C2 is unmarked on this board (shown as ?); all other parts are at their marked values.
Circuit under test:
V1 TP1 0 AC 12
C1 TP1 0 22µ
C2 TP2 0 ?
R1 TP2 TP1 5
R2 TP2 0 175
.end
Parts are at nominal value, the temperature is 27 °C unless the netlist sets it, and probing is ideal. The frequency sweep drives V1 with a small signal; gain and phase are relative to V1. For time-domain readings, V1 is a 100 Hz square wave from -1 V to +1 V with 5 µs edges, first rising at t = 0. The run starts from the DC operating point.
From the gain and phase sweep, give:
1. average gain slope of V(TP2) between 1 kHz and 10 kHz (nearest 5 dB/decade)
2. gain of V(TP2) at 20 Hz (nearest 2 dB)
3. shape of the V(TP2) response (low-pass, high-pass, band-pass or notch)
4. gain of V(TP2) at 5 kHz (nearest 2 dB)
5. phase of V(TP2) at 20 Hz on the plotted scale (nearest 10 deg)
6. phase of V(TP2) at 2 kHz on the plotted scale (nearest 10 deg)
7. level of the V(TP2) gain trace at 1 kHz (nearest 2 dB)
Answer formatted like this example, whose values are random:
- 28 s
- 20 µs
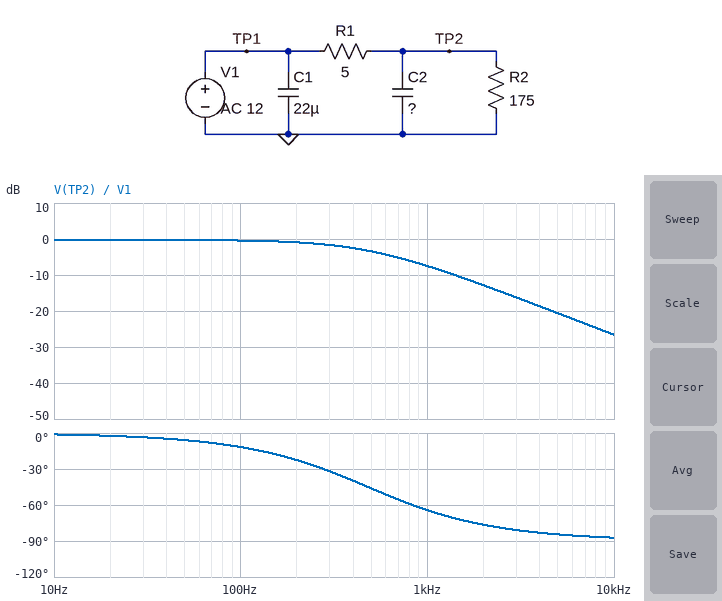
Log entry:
- -20 dB/decade
- 0 dB
- low-pass
- -20 dB
- 0 deg
- -80 deg
- -8 dB
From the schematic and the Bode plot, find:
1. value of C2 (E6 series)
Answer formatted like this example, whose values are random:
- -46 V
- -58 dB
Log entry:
- 68 µF
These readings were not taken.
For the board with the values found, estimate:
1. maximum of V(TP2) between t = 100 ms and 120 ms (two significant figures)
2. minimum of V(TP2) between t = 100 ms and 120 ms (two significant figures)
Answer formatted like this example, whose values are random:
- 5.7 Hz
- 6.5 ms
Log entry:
- 970 mV
- -970 mV
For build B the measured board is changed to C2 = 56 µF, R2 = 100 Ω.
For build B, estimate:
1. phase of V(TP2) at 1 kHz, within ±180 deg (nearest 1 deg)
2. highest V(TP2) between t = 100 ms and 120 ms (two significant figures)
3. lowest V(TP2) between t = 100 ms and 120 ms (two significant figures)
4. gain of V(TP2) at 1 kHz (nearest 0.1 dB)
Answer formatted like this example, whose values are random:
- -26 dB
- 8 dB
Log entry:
- -59 deg
- 950 mV
- -950 mV
- -6.2 dB
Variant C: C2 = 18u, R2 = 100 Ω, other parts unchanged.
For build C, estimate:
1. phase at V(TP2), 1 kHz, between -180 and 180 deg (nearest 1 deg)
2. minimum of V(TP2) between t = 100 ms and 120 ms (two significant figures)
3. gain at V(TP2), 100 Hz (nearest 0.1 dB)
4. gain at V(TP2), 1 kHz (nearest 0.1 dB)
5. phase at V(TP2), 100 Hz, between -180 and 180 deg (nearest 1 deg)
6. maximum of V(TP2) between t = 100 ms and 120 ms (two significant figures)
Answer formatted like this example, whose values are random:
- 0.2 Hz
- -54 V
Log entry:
- -28 deg
- -950 mV
- -0.4 dB
- -1.5 dB
- -3 deg
- 950 mV
